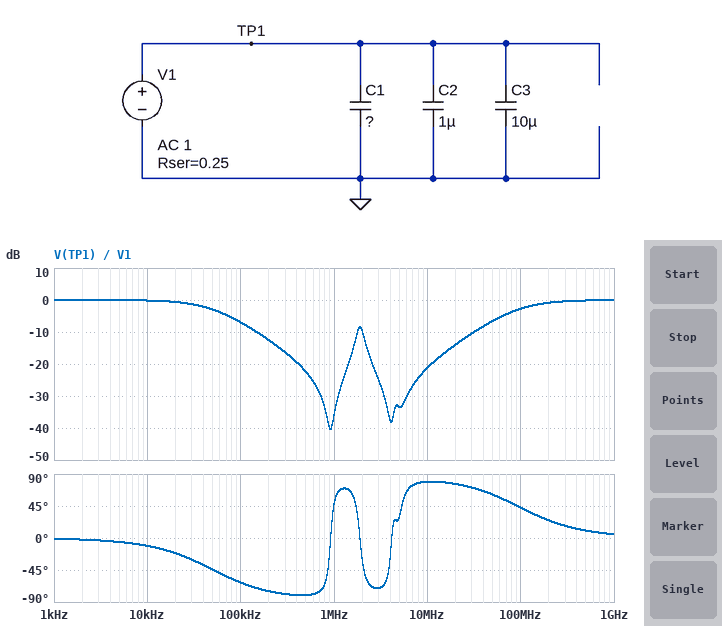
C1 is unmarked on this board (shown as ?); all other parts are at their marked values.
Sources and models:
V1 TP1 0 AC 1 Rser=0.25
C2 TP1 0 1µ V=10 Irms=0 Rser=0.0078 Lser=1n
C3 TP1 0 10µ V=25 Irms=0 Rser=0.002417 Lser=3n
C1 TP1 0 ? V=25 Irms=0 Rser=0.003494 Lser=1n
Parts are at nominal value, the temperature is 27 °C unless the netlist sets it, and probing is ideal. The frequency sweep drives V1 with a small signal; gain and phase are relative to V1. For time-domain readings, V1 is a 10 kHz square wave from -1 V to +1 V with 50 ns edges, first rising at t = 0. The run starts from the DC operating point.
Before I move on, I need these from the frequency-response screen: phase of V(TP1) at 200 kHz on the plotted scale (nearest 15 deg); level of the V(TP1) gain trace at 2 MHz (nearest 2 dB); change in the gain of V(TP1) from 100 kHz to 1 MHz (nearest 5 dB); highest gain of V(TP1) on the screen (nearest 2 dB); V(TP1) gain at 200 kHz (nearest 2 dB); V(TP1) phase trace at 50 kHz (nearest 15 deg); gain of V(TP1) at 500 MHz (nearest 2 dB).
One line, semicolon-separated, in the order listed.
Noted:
-75 deg; -10 dB; -30 dB; 0 dB; -12 dB; -45 deg; 0 dB
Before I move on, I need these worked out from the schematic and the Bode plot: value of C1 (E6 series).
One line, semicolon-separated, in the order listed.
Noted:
1.5 µF
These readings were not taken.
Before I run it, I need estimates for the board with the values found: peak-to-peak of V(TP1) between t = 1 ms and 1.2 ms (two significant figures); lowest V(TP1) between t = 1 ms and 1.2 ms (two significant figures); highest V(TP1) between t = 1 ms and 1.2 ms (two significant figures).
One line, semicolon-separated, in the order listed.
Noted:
2.0 V; -1.0 V; 1.0 V
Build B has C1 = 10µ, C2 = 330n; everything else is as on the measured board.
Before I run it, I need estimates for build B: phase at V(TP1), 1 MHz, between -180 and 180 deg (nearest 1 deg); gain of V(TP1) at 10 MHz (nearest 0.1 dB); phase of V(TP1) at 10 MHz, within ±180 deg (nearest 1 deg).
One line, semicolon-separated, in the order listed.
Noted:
28 deg; -26.2 dB; 66 deg
